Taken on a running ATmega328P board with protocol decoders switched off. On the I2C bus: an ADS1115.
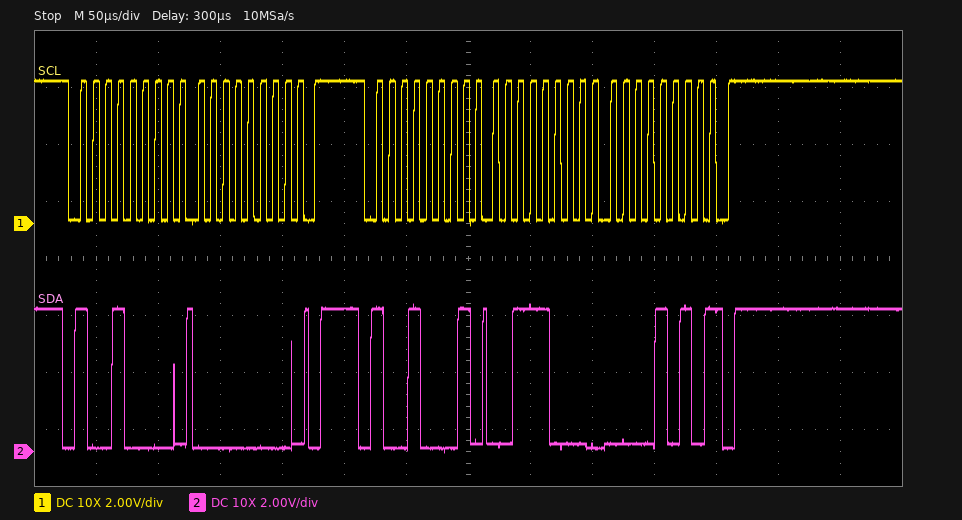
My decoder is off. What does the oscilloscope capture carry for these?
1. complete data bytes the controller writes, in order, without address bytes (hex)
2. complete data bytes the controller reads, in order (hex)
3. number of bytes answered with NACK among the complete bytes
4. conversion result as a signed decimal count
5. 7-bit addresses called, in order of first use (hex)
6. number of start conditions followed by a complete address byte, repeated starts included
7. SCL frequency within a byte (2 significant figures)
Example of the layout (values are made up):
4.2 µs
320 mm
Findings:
00
38 0A
1
14346
0x48
2
100 kHz
